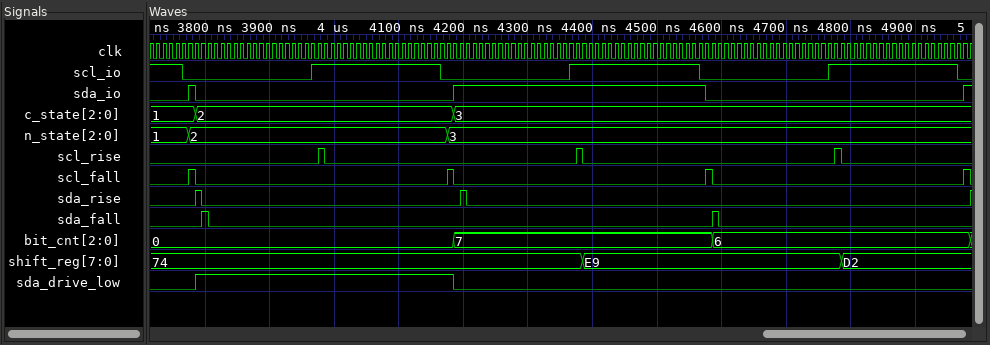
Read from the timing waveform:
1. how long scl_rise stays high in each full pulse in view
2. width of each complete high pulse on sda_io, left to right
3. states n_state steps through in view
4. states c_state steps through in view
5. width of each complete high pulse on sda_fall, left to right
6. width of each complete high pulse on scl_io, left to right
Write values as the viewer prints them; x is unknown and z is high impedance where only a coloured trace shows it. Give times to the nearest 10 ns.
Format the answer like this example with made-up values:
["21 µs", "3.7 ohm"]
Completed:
["10 ns, 10 ns, 10 ns", "10 ns, 390 ns", "1, 2, 3", "1, 2, 3", "10 ns, 10 ns", "200 ns, 200 ns, 200 ns"]
